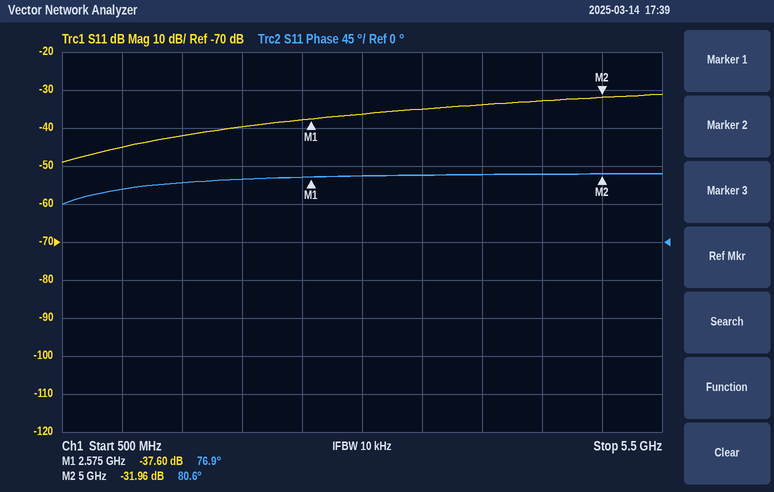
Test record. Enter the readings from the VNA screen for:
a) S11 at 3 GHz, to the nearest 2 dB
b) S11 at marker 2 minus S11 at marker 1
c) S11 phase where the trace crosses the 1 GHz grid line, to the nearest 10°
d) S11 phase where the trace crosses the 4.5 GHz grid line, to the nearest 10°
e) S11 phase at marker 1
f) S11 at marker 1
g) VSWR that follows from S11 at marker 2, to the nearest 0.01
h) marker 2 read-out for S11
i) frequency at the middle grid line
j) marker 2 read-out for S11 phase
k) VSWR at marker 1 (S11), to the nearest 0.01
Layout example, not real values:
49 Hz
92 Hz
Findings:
-36 dB
5.64 dB
60°
80°
76.9°
-37.60 dB
1.05
-31.96 dB
3 GHz
80.6°
1.03
